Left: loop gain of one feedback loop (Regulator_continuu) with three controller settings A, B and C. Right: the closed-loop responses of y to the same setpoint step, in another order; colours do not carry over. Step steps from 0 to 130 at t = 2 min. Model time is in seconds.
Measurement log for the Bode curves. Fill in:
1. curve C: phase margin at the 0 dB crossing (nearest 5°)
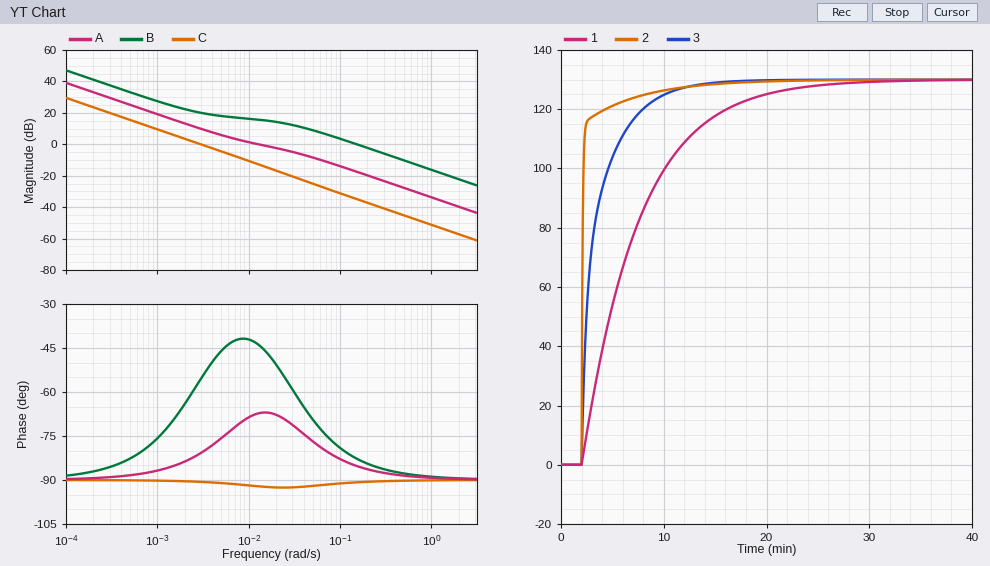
90°
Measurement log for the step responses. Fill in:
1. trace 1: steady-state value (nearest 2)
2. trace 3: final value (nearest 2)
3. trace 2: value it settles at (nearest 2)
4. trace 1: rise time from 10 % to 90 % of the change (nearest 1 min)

130
130
130
12 min
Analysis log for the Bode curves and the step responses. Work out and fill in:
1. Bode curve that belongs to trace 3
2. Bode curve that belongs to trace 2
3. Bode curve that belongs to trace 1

A
B
C
